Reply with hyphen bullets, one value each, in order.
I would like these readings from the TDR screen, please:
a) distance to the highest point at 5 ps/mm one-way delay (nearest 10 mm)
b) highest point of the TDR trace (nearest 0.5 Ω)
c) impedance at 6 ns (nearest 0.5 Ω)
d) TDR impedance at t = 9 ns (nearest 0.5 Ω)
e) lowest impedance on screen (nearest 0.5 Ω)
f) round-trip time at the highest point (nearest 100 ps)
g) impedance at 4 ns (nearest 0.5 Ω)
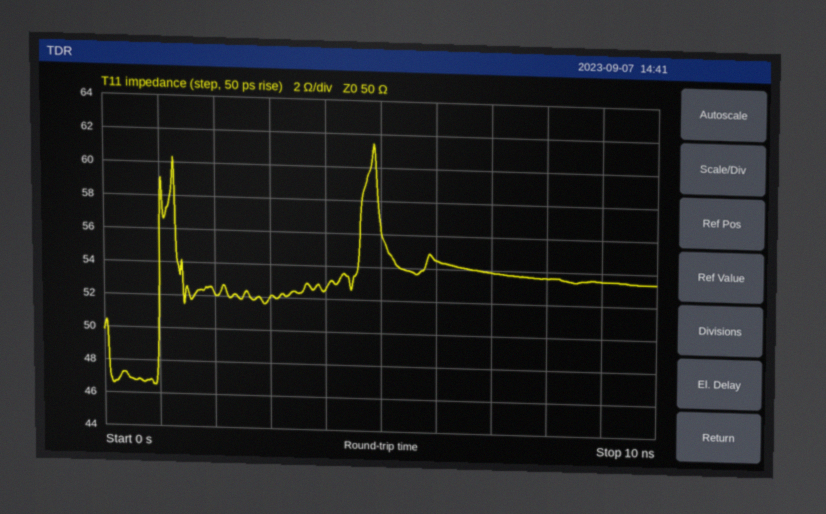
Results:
- 490 mm
- 61.5 Ω
- 54.5 Ω
- 53.5 Ω
- 46.5 Ω
- 4.9 ns
- 52.5 Ω
